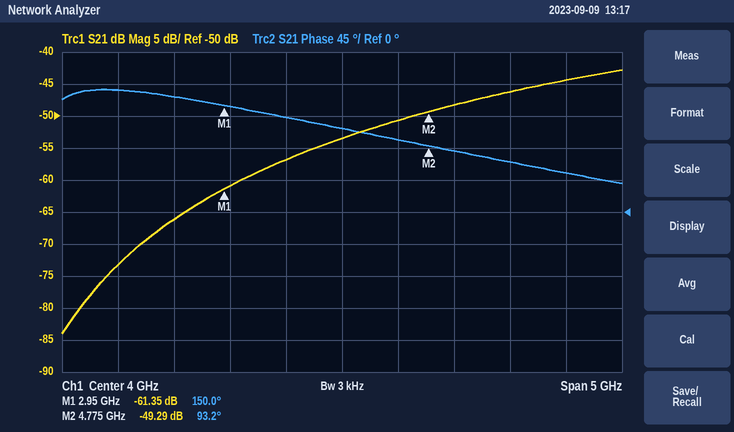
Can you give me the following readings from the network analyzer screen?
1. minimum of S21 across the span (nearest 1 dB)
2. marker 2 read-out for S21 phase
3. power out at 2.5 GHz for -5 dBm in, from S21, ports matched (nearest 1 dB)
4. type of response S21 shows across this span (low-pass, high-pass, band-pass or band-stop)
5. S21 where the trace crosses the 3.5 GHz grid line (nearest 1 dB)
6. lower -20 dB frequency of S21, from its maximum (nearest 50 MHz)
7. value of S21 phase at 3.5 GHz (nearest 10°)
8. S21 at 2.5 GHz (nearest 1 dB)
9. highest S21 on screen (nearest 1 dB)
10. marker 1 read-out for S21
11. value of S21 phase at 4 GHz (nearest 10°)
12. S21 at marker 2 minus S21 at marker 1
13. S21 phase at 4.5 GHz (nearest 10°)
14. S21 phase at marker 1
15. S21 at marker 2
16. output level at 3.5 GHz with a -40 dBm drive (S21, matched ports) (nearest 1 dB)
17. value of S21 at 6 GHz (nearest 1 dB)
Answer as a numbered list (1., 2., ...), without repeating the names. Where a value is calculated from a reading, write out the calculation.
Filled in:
1. -84 dB
2. 93.2°
3. -5 dBm + (-66 dB) = -71 dBm
4. high-pass
5. -57 dB
6. 2.80 GHz
7. 130°
8. -66 dB
9. -43 dB
10. -61.35 dB
11. 120°
12. -49.29 − (-61.35) = 12.06 dB
13. 100°
14. 150.0°
15. -49.29 dB
16. -40 dBm + (-57 dB) = -97 dBm
17. -44 dB
